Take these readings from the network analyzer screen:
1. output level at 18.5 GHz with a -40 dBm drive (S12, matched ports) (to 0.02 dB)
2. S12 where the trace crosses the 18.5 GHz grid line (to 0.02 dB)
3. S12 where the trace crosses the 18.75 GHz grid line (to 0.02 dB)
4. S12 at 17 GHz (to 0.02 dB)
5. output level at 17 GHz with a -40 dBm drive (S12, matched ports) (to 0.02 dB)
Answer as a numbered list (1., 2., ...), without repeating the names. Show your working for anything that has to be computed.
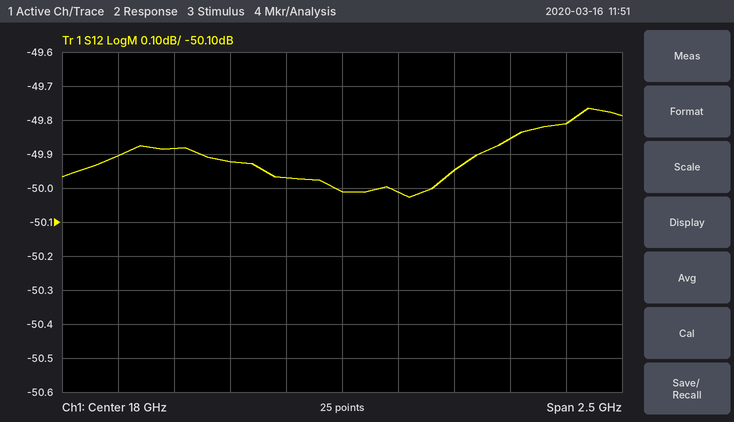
1. -40 dBm + (-49.94 dB) = -89.94 dBm
2. -49.94 dB
3. -49.86 dB
4. -49.90 dB
5. -40 dBm + (-49.90 dB) = -89.90 dBm
